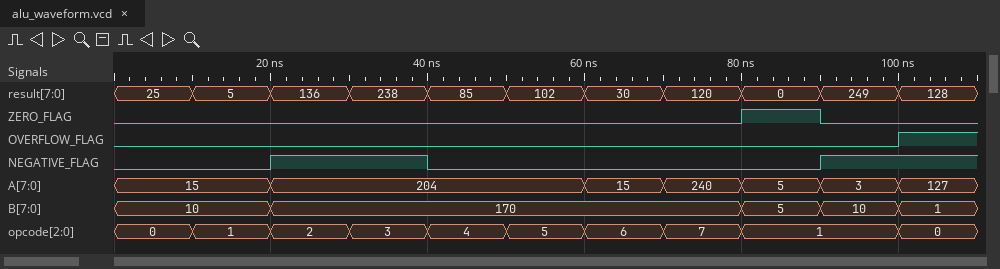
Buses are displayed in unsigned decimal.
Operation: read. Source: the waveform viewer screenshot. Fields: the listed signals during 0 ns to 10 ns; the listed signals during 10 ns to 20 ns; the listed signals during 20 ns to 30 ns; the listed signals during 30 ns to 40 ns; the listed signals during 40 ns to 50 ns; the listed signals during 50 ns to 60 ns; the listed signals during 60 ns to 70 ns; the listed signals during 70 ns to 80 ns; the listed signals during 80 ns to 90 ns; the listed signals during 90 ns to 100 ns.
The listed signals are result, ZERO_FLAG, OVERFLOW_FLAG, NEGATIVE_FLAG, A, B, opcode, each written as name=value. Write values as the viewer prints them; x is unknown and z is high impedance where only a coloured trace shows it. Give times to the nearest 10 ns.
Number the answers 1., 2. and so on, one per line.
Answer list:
1. result=25, ZERO_FLAG=0, OVERFLOW_FLAG=0, NEGATIVE_FLAG=0, A=15, B=10, opcode=0
2. result=5, ZERO_FLAG=0, OVERFLOW_FLAG=0, NEGATIVE_FLAG=0, A=15, B=10, opcode=1
3. result=136, ZERO_FLAG=0, OVERFLOW_FLAG=0, NEGATIVE_FLAG=1, A=204, B=170, opcode=2
4. result=238, ZERO_FLAG=0, OVERFLOW_FLAG=0, NEGATIVE_FLAG=1, A=204, B=170, opcode=3
5. result=85, ZERO_FLAG=0, OVERFLOW_FLAG=0, NEGATIVE_FLAG=0, A=204, B=170, opcode=4
6. result=102, ZERO_FLAG=0, OVERFLOW_FLAG=0, NEGATIVE_FLAG=0, A=204, B=170, opcode=5
7. result=30, ZERO_FLAG=0, OVERFLOW_FLAG=0, NEGATIVE_FLAG=0, A=15, B=170, opcode=6
8. result=120, ZERO_FLAG=0, OVERFLOW_FLAG=0, NEGATIVE_FLAG=0, A=240, B=170, opcode=7
9. result=0, ZERO_FLAG=1, OVERFLOW_FLAG=0, NEGATIVE_FLAG=0, A=5, B=5, opcode=1
10. result=249, ZERO_FLAG=0, OVERFLOW_FLAG=0, NEGATIVE_FLAG=1, A=3, B=10, opcode=1
